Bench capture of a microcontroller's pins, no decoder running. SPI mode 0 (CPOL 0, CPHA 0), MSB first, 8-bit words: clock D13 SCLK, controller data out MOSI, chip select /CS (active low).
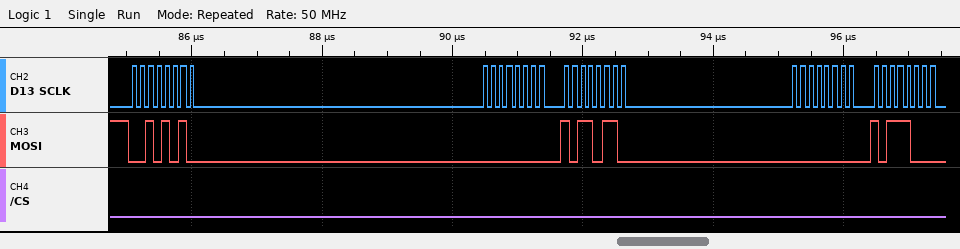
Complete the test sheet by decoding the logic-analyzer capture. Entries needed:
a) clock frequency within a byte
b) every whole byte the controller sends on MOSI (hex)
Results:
8 MHz
0x2A 0x00 0xB6 0x00 0xB8
